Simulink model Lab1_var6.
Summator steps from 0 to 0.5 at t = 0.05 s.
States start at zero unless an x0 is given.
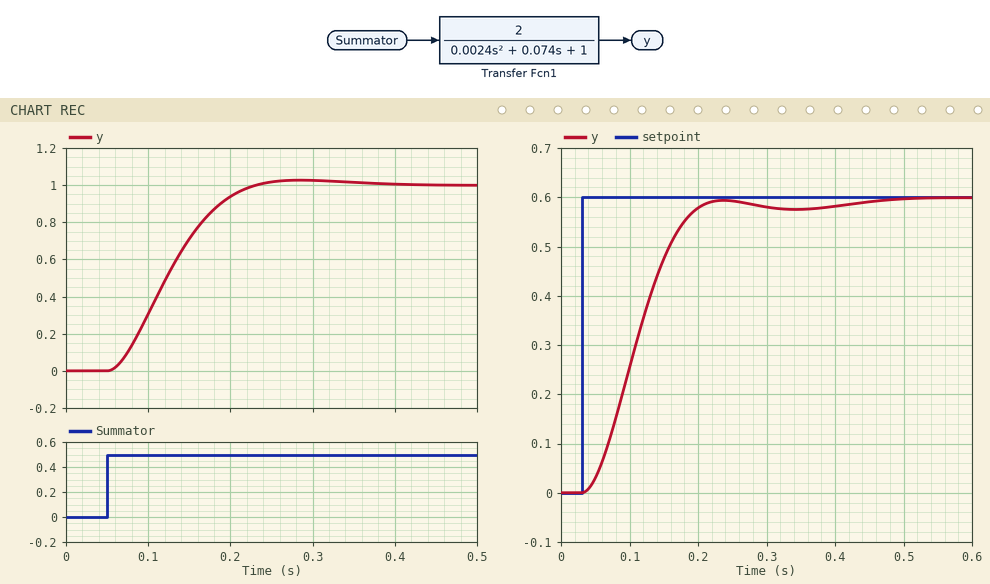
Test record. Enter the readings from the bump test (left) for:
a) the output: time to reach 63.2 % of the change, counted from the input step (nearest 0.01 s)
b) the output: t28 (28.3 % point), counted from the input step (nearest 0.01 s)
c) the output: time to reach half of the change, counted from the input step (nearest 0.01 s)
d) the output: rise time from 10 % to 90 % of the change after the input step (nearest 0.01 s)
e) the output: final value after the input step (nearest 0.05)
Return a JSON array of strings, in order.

["0.09 s", "0.05 s", "0.07 s", "0.11 s", "1.00"]
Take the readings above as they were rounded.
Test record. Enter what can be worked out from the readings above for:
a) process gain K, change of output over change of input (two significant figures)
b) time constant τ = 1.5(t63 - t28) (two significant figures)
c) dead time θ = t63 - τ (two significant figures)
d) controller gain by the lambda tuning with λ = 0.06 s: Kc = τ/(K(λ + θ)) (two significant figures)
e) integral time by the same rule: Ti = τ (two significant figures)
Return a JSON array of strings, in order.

["2.0", "0.060 s", "0.030 s", "0.33", "0.060 s"]
